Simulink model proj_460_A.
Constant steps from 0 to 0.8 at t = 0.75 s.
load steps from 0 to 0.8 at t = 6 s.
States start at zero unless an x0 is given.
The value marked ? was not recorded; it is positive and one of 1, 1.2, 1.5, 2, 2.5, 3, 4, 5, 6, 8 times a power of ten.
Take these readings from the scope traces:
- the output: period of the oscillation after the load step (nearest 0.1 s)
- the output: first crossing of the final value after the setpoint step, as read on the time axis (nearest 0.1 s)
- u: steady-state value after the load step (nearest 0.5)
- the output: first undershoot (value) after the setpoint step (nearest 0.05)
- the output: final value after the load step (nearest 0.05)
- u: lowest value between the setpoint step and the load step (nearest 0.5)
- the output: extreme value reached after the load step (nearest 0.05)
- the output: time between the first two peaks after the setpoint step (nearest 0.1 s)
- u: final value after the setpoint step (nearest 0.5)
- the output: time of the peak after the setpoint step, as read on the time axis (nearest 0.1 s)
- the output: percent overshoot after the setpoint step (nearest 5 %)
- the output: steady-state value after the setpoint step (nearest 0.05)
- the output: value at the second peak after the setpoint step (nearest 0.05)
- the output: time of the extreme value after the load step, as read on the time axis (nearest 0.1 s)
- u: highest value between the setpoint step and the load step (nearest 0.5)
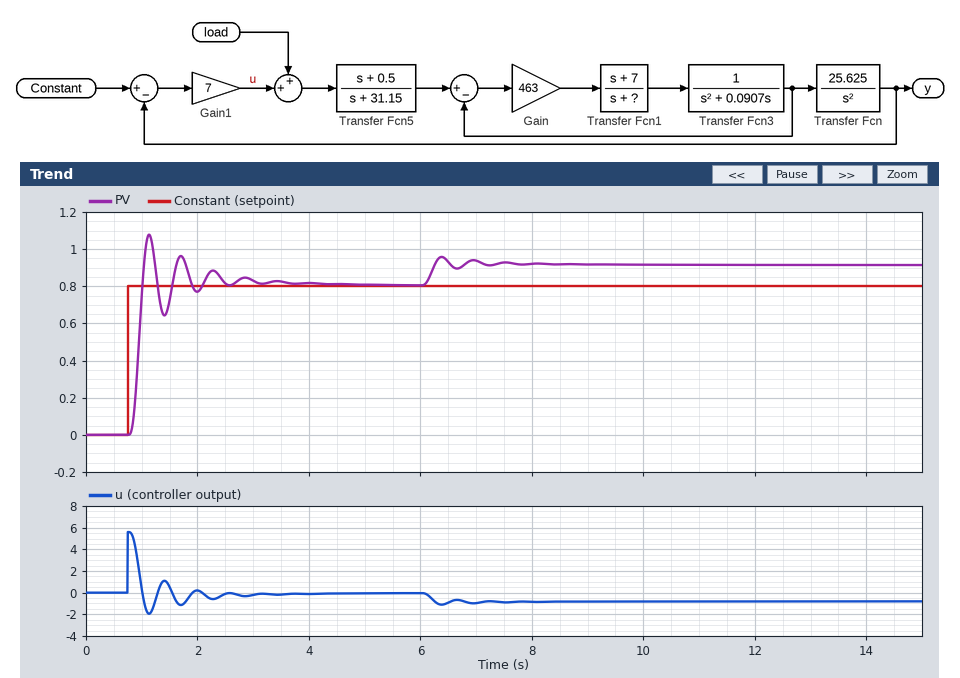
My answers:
0.6 s
1.0 s
-1.0
0.65
0.90
-2.0
0.95
0.6 s
0.0
1.1 s
35 %
0.80
0.95
6.4 s
5.5
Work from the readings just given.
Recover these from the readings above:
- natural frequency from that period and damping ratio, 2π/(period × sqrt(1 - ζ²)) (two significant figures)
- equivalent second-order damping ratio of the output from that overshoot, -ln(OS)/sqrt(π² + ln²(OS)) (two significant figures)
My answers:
11 rad/s
0.32
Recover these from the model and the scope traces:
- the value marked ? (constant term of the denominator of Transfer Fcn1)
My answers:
40
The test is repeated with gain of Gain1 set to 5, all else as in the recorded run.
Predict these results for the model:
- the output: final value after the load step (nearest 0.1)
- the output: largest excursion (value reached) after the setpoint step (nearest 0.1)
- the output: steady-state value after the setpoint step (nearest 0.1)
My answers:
1.0
0.9
0.8
